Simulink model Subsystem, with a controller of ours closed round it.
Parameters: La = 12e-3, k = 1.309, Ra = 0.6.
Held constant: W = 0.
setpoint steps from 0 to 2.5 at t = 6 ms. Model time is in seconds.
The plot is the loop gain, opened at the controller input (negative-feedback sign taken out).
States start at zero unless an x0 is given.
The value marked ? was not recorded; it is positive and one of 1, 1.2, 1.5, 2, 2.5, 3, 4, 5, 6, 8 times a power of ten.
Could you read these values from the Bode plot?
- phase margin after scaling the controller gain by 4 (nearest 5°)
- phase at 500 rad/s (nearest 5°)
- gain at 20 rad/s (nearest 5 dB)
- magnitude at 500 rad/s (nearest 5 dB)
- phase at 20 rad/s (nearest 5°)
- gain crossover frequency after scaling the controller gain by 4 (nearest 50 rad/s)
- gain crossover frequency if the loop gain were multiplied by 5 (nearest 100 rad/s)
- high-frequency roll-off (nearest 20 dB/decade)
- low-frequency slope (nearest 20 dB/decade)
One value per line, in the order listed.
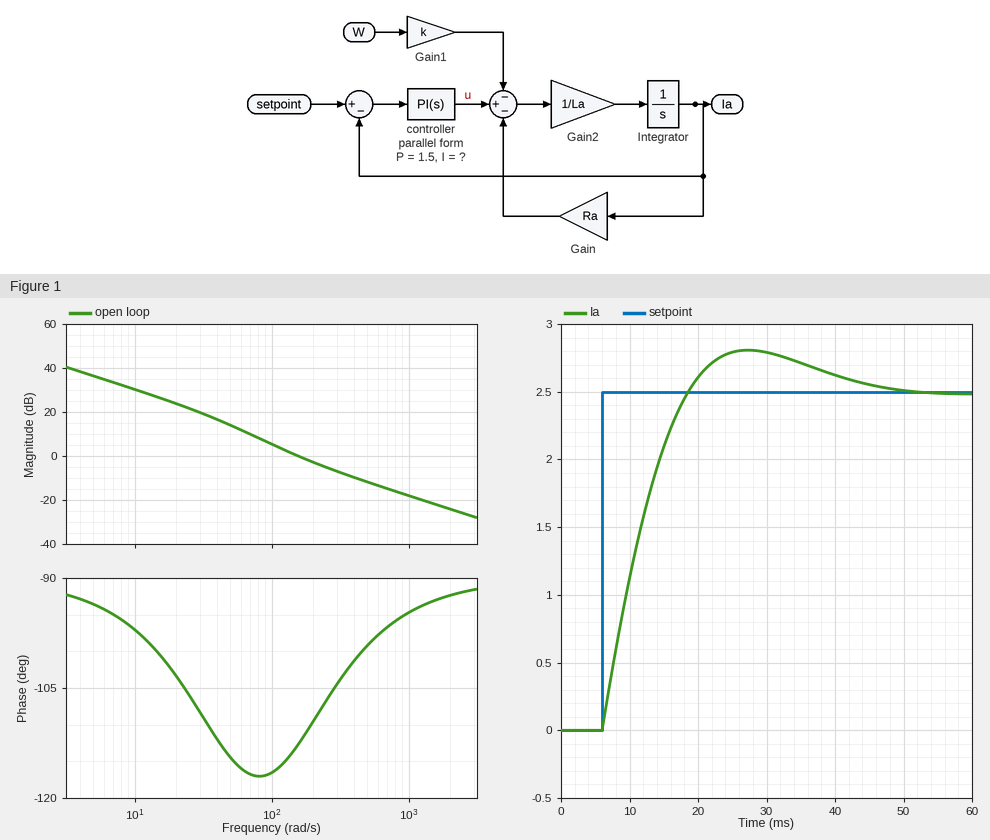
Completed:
80°
-100°
25 dB
-10 dB
-105°
500 rad/s
600 rad/s
-20 dB/decade
-20 dB/decade
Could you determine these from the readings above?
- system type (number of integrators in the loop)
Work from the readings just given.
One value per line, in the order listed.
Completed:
1
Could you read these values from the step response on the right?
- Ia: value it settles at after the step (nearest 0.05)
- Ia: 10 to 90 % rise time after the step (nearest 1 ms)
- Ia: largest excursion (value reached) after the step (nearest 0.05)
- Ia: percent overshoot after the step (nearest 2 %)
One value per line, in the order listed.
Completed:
2.50
9 ms
2.80
12 %
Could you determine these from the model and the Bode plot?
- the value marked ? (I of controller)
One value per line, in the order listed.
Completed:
200
